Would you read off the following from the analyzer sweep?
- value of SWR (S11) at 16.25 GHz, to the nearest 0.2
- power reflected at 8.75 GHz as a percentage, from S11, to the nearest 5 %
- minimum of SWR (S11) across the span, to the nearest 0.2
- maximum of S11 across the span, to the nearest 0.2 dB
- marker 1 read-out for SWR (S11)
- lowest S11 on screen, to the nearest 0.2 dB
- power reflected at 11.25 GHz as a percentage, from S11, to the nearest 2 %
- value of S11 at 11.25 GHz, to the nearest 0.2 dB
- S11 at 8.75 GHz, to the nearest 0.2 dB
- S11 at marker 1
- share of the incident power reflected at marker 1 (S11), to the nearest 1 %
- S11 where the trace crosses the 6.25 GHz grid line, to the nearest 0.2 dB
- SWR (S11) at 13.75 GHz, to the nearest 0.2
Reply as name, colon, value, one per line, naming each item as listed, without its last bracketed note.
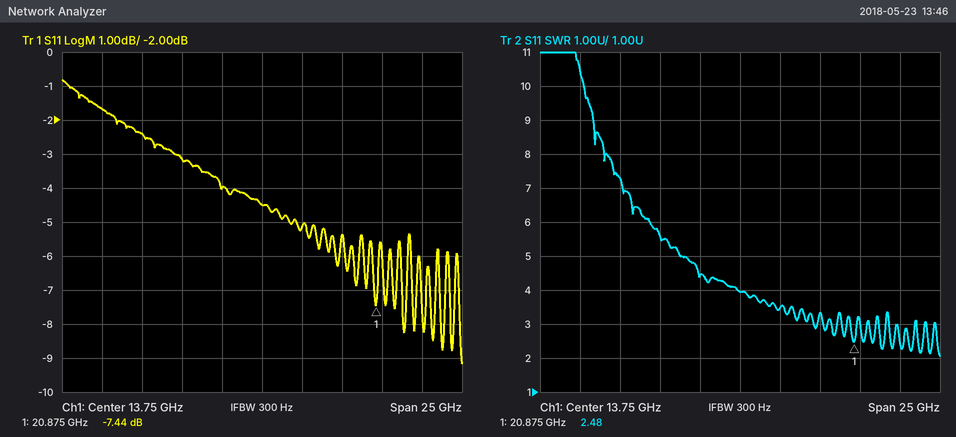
value of SWR (S11) at 16.25 GHz, to the nearest 0.2: 3.4
power reflected at 8.75 GHz as a percentage, from S11, to the nearest 5 %: 50 %
minimum of SWR (S11) across the span, to the nearest 0.2: 2.0
maximum of S11 across the span, to the nearest 0.2 dB: -0.8 dB
marker 1 read-out for SWR: 2.48
lowest S11 on screen, to the nearest 0.2 dB: -9.2 dB
power reflected at 11.25 GHz as a percentage, from S11, to the nearest 2 %: 40 %
value of S11 at 11.25 GHz, to the nearest 0.2 dB: -4.0 dB
S11 at 8.75 GHz, to the nearest 0.2 dB: -3.2 dB
S11 at marker 1: -7.44 dB
share of the incident power reflected at marker 1 (S11), to the nearest 1 %: 18 %
S11 where the trace crosses the 6.25 GHz grid line, to the nearest 0.2 dB: -2.4 dB
SWR (S11) at 13.75 GHz, to the nearest 0.2: 4.0
